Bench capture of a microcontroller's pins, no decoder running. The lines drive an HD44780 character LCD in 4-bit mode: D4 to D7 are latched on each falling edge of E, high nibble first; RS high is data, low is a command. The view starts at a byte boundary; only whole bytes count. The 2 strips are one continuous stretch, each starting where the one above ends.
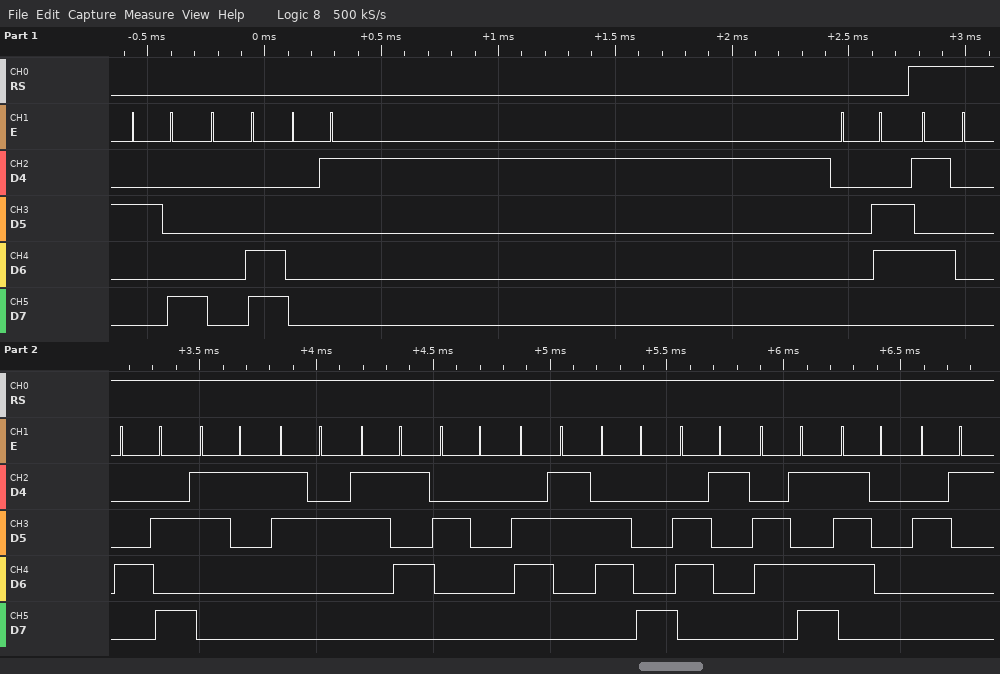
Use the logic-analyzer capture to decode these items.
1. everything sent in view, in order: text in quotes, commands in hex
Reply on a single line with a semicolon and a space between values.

0x28 0x0C 0x01 0x06 "PJ125 champ!"
